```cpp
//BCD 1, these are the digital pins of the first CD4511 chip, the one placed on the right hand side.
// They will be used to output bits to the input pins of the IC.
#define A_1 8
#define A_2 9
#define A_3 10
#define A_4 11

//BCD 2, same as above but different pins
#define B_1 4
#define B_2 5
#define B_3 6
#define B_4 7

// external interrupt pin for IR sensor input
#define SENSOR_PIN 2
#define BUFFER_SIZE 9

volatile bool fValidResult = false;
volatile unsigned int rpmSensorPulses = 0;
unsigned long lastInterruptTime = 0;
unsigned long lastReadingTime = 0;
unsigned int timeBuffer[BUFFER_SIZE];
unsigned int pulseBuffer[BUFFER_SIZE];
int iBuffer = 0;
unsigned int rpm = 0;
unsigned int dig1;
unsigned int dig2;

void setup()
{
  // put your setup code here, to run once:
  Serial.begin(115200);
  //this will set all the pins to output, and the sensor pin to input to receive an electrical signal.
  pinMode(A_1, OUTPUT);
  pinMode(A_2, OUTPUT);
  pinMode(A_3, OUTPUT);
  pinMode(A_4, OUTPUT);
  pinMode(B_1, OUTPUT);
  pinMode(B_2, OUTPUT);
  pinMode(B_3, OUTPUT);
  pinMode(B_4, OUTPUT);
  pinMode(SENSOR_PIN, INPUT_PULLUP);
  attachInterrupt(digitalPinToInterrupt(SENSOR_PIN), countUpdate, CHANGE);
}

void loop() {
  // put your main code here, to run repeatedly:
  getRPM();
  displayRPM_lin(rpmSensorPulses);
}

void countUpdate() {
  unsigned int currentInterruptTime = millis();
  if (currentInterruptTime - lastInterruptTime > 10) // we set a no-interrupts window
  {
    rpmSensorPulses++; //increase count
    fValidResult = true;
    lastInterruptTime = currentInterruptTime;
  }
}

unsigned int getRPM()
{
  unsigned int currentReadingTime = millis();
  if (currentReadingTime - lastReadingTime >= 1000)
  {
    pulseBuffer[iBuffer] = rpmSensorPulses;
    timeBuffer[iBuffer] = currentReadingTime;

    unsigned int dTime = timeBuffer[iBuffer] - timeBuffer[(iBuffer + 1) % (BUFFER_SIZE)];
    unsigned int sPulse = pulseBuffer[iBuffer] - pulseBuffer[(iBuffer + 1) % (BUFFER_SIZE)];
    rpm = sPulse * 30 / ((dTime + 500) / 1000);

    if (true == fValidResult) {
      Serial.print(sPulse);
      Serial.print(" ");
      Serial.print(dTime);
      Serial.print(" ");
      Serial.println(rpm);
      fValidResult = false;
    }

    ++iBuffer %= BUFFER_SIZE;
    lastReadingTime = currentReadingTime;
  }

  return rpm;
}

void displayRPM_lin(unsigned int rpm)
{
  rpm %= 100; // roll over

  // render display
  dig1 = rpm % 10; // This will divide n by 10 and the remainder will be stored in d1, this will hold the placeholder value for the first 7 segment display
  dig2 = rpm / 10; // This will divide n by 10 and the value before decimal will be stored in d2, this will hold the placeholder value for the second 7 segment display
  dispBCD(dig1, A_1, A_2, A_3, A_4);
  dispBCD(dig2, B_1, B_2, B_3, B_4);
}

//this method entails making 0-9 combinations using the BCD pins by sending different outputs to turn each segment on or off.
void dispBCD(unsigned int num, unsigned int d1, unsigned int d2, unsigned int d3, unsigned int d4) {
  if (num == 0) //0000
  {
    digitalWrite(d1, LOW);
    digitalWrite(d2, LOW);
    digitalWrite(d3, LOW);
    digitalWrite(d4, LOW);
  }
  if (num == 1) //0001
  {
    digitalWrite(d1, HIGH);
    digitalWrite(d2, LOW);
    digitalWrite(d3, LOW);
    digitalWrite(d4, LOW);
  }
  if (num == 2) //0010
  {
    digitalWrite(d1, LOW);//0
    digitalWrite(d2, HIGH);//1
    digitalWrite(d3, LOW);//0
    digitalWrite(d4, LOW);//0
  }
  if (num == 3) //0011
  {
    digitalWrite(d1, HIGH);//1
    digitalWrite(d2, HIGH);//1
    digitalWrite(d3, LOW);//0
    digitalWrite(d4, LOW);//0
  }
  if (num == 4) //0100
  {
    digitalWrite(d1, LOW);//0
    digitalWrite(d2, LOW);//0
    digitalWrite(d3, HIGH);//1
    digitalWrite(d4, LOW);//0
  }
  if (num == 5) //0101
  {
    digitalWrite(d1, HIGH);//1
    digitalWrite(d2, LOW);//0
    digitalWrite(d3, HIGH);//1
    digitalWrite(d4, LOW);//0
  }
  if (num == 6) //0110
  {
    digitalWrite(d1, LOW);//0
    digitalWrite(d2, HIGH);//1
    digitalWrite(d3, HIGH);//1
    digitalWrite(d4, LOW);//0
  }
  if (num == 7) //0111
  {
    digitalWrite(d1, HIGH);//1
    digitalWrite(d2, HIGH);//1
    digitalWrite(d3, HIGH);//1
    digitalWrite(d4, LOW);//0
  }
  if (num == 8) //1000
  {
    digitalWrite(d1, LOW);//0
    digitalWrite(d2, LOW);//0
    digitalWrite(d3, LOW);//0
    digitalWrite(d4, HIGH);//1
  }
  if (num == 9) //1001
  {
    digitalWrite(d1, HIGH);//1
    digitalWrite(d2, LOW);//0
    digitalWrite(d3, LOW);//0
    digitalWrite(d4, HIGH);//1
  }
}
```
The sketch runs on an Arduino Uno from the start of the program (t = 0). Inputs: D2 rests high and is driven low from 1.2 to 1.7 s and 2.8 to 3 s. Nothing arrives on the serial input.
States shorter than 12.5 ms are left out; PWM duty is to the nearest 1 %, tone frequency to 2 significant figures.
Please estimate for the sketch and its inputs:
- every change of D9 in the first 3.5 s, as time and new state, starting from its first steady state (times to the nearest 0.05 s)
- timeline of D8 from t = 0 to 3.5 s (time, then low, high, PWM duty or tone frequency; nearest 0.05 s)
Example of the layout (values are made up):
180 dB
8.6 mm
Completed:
0 s low; 1.7 s high; 3 s low
0 s low; 1.2 s high; 1.7 s low; 2.8 s high; 3 s low
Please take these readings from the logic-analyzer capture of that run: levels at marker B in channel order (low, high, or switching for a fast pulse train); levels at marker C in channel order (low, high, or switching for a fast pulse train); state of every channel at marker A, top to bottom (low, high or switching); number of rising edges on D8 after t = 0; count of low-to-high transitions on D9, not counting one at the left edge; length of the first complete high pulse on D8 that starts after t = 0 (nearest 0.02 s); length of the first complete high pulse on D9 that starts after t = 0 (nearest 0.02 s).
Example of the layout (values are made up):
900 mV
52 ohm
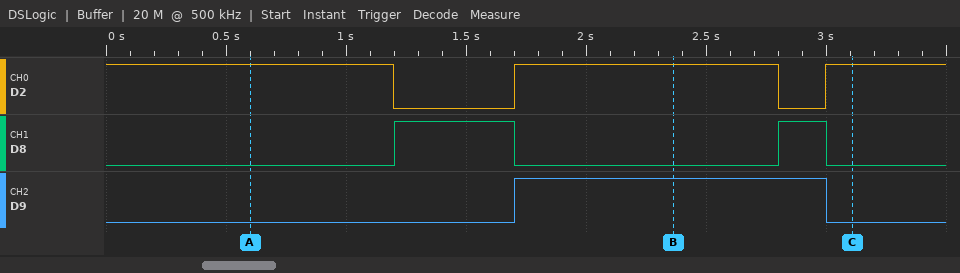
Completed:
D2 high, D8 low, D9 high
D2 high, D8 low, D9 low
D2 high, D8 low, D9 low
2
1
0.50 s
1.30 s
